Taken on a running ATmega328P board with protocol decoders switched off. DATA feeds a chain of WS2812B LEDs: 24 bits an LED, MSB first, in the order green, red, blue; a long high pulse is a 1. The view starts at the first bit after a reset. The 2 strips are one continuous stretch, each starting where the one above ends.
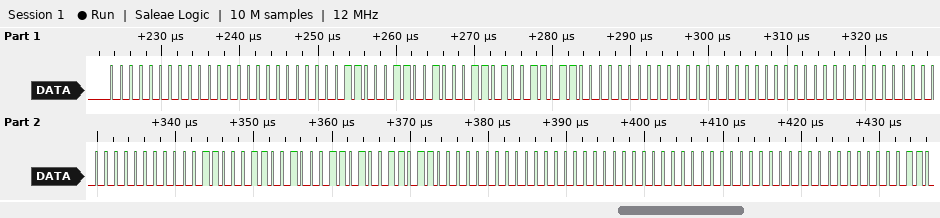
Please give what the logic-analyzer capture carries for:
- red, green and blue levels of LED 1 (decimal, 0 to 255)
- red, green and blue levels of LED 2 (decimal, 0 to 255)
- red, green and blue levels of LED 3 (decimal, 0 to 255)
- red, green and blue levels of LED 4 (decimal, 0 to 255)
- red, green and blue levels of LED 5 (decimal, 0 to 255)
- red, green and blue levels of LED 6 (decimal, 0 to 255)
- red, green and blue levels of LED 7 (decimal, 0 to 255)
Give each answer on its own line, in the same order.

0, 0, 0
70, 198, 155
0, 0, 0
0, 0, 0
70, 198, 155
0, 0, 0
0, 0, 0
